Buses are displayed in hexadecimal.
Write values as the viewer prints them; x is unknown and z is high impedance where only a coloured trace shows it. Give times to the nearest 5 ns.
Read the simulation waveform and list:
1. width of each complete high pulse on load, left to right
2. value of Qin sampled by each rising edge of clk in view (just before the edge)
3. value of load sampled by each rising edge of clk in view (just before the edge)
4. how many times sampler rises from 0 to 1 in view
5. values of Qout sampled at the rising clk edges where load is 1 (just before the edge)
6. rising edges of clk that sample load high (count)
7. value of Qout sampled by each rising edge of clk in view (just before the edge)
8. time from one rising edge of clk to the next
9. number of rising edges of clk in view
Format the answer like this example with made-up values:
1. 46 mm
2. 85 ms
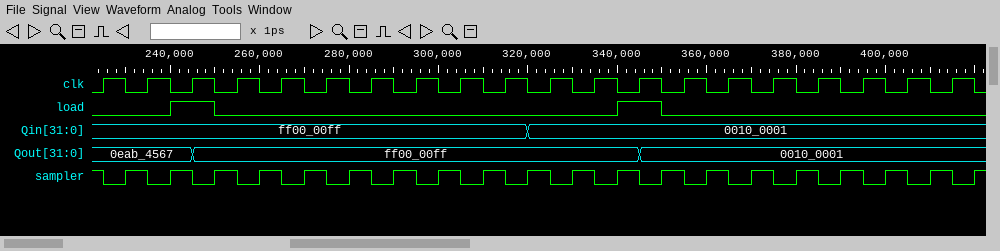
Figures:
1. 10 ns, 10 ns
2. ff00_00ff, ff00_00ff, ff00_00ff, ff00_00ff, ff00_00ff, ff00_00ff, ff00_00ff, ff00_00ff, ff00_00ff, ff00_00ff, 0010_0001, 0010_0001, 0010_0001, 0010_0001, 0010_0001, 0010_0001, 0010_0001, 0010_0001, 0010_0001, 0010_0001
3. 0 0 1 0 0 0 0 0 0 0 0 0 1 0 0 0 0 0 0 0
4. 20
5. 0eab_4567, ff00_00ff
6. 2
7. 0eab_4567, 0eab_4567, 0eab_4567, ff00_00ff, ff00_00ff, ff00_00ff, ff00_00ff, ff00_00ff, ff00_00ff, ff00_00ff, ff00_00ff, ff00_00ff, ff00_00ff, 0010_0001, 0010_0001, 0010_0001, 0010_0001, 0010_0001, 0010_0001, 0010_0001
8. 10 ns
9. 20
